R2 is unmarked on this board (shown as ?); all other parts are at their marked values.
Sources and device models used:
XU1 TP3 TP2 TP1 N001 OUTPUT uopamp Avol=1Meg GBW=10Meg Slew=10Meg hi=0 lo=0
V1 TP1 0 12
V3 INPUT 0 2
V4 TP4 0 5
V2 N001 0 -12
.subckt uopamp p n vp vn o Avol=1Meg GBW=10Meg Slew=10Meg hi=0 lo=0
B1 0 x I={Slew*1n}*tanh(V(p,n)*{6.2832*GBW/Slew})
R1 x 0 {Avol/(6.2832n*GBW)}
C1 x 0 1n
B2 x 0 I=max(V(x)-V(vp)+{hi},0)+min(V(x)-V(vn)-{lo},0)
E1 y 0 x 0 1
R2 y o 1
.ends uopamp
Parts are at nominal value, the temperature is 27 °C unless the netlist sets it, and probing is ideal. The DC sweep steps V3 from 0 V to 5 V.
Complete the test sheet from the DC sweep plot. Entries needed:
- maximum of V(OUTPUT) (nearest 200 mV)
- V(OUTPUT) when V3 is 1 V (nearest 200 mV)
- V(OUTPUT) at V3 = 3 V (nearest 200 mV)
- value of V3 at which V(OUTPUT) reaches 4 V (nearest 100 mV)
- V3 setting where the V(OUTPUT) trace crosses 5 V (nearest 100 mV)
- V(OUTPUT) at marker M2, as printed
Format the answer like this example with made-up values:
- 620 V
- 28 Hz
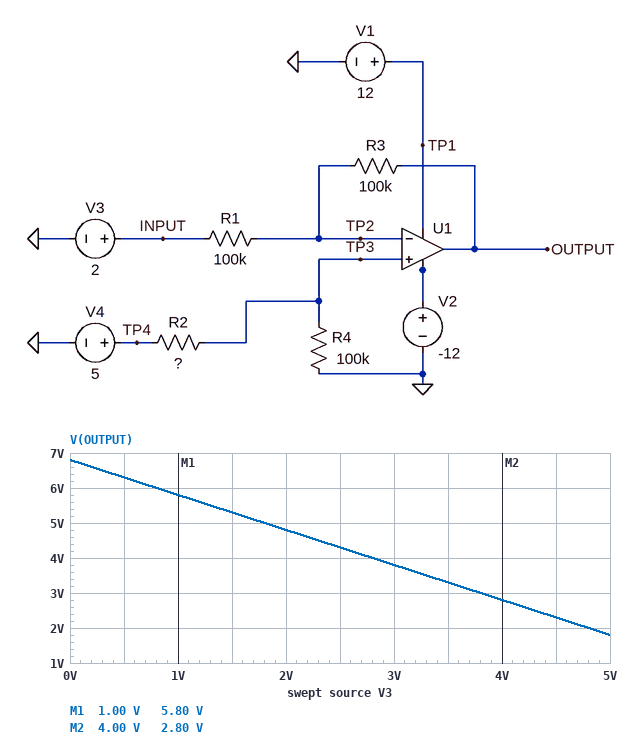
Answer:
- 6.8 V
- 5.8 V
- 3.8 V
- 2.8 V
- 1.8 V
- 2.80 V
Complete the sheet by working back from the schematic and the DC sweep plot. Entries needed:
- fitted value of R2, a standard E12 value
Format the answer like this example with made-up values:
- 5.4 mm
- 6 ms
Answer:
- 47 kΩ
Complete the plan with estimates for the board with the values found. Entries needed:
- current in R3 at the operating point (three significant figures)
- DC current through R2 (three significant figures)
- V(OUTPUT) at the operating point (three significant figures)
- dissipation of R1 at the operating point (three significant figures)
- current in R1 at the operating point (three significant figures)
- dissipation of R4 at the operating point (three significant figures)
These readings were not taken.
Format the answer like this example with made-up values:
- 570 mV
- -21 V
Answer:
- 14.0 µA
- 34.0 µA
- 4.80 V
- 19.6 µW
- 14.0 µA
- 116 µW
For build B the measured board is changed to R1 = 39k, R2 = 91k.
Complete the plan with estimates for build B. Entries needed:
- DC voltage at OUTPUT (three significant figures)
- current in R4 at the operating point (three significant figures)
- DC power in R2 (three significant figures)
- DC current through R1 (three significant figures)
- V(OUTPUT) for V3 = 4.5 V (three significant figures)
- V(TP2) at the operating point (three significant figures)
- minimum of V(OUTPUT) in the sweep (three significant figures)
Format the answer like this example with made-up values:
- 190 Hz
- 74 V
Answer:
- 4.20 V
- 26.2 µA
- 62.4 µW
- 15.8 µA
- -2.21 V
- 2.62 V
- -3.49 V
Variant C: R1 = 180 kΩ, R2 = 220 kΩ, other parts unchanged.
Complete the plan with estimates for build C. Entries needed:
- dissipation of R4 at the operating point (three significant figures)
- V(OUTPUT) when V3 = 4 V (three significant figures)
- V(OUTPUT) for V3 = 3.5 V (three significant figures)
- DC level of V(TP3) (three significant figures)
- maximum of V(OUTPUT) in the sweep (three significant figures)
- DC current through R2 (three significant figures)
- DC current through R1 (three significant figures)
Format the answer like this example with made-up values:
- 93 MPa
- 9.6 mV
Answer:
- 24.4 µW
- 208 mV
- 486 mV
- 1.56 V
- 2.43 V
- 15.6 µA
- 2.43 µA
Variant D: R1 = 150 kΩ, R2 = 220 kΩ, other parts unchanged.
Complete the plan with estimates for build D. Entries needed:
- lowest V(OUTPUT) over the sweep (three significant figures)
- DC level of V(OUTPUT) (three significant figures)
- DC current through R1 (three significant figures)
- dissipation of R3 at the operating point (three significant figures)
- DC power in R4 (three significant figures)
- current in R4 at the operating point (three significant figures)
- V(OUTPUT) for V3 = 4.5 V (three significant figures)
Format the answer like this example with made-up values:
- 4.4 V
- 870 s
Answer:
- -729 mV
- 1.27 V
- 2.92 µA
- 851 nW
- 24.4 µW
- 15.6 µA
- -396 mV
